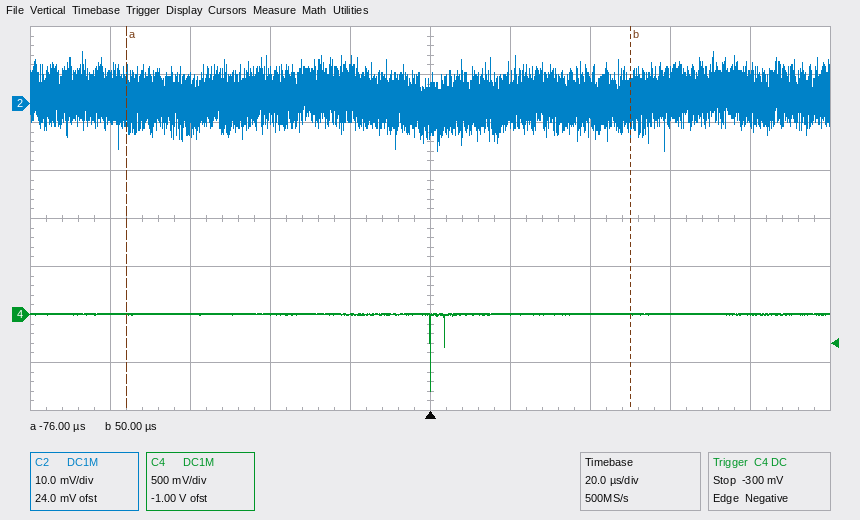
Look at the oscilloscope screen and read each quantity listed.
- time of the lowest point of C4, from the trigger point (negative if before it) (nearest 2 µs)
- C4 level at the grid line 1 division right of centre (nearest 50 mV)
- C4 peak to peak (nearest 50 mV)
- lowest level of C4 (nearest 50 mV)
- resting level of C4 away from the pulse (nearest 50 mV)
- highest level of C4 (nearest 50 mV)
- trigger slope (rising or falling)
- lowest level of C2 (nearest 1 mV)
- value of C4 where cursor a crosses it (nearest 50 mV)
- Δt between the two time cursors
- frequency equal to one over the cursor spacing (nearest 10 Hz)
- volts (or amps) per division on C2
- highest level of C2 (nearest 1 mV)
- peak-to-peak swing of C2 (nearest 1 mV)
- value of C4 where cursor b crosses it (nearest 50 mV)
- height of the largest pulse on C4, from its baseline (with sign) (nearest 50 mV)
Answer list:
0 µs
0 mV
800 mV
-800 mV
0 mV
0 mV
falling
-10 mV
0 mV
126 µs
7.94 kHz
10 mV
11 mV
21 mV
0 mV
-800 mV
